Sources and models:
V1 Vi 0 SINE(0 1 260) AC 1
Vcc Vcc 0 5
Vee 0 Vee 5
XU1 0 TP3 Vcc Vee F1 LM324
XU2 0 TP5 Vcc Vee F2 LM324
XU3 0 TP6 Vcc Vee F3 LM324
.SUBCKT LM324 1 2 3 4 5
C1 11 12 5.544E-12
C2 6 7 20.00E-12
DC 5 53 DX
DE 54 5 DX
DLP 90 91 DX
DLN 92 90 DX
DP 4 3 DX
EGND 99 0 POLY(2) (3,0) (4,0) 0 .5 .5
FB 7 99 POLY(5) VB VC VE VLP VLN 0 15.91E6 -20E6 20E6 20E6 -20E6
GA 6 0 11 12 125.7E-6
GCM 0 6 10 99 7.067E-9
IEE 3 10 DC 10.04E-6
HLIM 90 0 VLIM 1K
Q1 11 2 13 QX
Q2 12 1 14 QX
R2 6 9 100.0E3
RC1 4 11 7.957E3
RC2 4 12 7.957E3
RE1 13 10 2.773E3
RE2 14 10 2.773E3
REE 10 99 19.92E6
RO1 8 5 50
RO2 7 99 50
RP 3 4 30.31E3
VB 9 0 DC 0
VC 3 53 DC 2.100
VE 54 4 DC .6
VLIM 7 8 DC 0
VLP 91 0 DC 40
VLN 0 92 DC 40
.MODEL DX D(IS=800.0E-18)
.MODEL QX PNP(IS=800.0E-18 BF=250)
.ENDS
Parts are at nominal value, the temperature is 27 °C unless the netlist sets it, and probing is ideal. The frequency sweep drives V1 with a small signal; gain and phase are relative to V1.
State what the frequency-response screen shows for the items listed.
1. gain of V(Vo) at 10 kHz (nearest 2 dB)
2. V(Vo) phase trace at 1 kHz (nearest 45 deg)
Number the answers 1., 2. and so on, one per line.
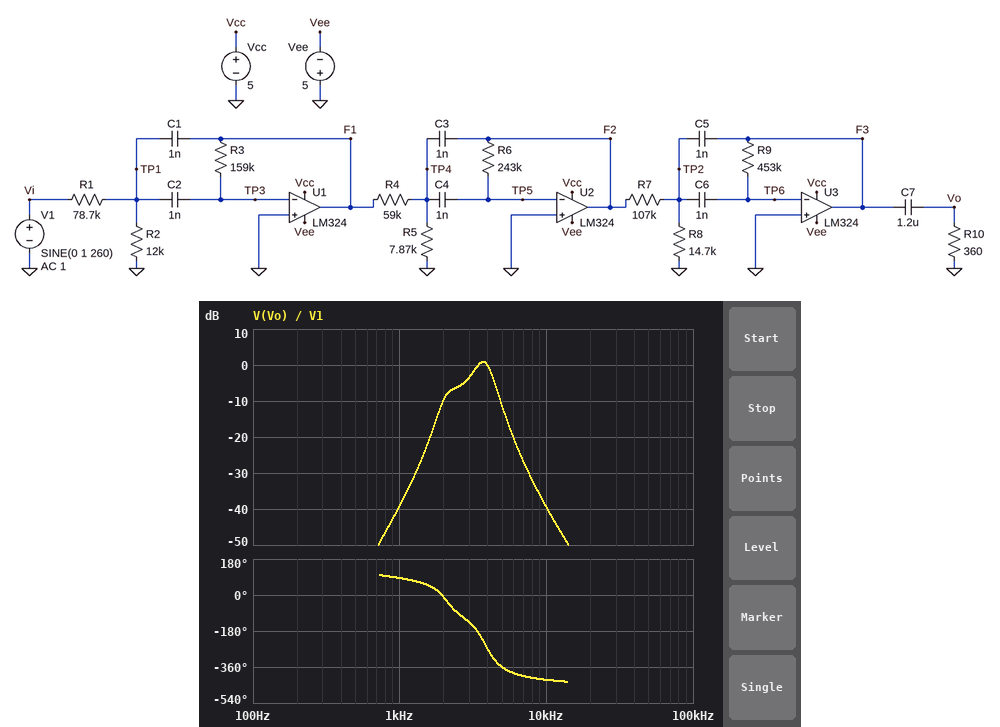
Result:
1. -40 dB
2. 90 deg
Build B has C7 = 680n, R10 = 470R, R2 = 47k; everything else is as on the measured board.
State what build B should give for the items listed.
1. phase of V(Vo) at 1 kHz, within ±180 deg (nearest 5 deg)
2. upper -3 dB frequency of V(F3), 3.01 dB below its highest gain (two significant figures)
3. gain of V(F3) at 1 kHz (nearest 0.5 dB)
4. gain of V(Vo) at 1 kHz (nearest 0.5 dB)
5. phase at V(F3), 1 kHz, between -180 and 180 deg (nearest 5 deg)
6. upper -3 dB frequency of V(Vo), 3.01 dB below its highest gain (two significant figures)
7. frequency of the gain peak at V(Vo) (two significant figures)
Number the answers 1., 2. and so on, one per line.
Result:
1. 75 deg
2. 3.5 kHz
3. -29.0 dB
4. -30.0 dB
5. 50 deg
6. 3.6 kHz
7. 2.2 kHz
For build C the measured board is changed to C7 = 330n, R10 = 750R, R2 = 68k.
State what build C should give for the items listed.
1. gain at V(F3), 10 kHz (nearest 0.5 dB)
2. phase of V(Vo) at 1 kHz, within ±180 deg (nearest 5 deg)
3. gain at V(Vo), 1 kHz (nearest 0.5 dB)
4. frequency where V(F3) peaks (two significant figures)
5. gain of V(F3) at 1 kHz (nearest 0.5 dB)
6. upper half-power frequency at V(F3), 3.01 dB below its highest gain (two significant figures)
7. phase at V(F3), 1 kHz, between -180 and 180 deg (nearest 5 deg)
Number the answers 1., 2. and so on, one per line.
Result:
1. -40.5 dB
2. 75 deg
3. -28.5 dB
4. 2.2 kHz
5. -27.0 dB
6. 2.9 kHz
7. 40 deg
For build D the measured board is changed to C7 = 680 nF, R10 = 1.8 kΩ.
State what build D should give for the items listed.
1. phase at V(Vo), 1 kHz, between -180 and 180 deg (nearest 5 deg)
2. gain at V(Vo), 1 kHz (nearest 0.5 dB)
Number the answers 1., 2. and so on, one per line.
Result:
1. 70 deg
2. -38.5 dB
